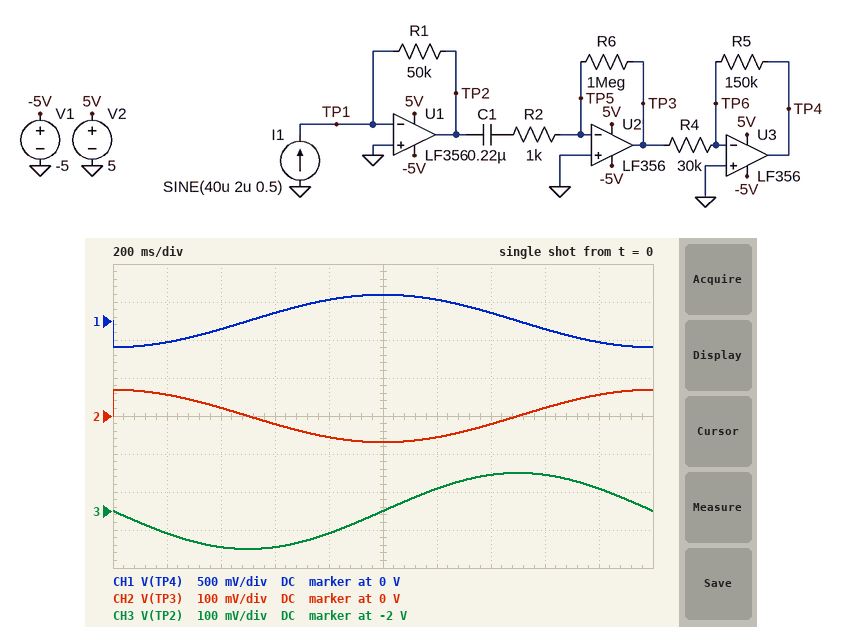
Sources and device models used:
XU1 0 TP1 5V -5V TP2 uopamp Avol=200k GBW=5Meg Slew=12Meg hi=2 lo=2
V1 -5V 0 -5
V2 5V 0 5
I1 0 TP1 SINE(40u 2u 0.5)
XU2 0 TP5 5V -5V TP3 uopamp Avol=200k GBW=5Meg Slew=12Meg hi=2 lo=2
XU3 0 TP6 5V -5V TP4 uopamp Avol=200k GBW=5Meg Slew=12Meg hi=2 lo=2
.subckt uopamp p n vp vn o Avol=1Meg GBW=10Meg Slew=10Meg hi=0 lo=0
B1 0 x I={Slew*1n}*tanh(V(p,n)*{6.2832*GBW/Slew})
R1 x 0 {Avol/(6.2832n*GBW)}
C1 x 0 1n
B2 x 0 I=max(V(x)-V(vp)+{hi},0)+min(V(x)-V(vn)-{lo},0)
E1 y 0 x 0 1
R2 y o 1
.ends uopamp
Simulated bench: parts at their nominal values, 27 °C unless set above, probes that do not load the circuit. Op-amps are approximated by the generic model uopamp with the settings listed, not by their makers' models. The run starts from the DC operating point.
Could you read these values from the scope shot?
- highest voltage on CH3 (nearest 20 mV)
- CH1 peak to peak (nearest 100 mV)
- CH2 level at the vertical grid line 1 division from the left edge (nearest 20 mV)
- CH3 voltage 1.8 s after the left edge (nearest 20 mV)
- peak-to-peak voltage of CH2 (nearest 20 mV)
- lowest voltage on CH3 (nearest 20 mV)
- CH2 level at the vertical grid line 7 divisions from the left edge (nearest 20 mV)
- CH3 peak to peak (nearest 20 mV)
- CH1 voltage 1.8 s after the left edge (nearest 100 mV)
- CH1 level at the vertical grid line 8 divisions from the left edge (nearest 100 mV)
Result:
-1.90 V
700 mV
60 mV
-1.94 V
140 mV
-2.10 V
-20 mV
200 mV
-300 mV
-100 mV
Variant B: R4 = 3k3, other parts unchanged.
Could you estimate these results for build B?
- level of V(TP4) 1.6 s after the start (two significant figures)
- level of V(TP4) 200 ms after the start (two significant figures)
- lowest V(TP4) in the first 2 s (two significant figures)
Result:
-970 mV
-2.5 V
-3.0 V
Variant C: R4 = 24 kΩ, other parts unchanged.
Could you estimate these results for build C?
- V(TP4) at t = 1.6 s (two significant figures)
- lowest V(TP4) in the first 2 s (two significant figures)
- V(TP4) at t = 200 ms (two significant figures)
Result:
-130 mV
-430 mV
-350 mV
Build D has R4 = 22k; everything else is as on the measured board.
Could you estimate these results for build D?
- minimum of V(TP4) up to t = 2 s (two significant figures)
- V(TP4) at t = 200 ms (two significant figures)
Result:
-470 mV
-380 mV
